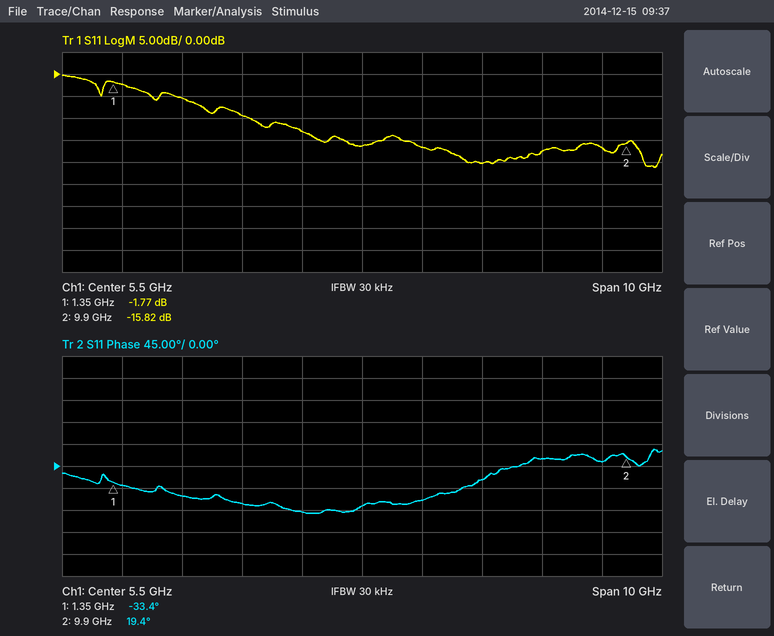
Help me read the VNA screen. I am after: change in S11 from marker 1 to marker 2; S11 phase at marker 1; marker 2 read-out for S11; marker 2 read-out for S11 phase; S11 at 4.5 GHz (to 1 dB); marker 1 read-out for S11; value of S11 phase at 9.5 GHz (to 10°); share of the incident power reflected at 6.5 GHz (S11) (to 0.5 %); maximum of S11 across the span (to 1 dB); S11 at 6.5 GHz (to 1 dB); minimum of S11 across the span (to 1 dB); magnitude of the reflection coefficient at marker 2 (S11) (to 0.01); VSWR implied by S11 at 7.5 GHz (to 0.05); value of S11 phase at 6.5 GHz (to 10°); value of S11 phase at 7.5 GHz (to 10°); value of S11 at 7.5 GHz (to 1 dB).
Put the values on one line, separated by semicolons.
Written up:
-14.05 dB; -33.4°; -15.82 dB; 19.4°; -13 dB; -1.77 dB; 10°; 2.0 %; 0 dB; -17 dB; -21 dB; 0.16; 1.20; -70°; -30°; -20 dB
